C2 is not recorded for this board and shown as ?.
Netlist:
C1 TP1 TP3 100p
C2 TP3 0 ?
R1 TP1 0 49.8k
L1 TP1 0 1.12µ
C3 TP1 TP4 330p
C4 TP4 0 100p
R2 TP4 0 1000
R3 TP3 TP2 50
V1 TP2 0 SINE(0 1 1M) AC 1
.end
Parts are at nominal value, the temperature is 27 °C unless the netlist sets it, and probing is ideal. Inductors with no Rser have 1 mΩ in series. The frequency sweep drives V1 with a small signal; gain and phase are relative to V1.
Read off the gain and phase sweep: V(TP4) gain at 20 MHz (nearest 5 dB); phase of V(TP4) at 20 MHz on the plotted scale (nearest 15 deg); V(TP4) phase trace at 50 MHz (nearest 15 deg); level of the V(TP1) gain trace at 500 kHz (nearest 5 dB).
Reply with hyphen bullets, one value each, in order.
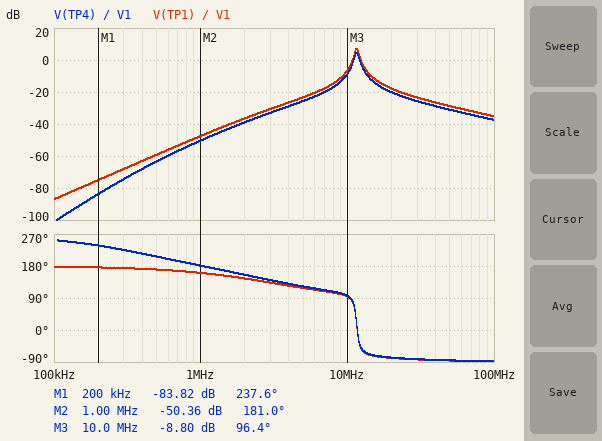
- -20 dB
- -75 deg
- -90 deg
- -60 dB
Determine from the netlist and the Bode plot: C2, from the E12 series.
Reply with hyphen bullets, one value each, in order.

- 1 nF
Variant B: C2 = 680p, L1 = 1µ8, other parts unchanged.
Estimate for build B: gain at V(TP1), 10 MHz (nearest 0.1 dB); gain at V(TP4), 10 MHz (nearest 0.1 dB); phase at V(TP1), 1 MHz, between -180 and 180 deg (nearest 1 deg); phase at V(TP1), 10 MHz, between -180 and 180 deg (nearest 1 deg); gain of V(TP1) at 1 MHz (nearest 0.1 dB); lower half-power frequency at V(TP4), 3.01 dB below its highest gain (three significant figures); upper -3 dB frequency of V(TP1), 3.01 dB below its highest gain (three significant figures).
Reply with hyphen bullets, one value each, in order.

- 2.3 dB
- 0 dB
- 166 deg
- -39 deg
- -43.1 dB
- 8.78 MHz
- 9.64 MHz
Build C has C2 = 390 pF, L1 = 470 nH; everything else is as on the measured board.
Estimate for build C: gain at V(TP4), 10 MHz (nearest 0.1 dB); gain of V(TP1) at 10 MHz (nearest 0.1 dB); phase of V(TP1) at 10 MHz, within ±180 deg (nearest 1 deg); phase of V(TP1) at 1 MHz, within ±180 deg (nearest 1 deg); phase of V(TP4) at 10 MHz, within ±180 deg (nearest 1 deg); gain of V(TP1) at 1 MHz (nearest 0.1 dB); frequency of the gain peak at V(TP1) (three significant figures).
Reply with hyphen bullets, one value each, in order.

- -19.1 dB
- -16.8 dB
- 120 deg
- 171 deg
- 122 deg
- -54.7 dB
- 18.4 MHz
